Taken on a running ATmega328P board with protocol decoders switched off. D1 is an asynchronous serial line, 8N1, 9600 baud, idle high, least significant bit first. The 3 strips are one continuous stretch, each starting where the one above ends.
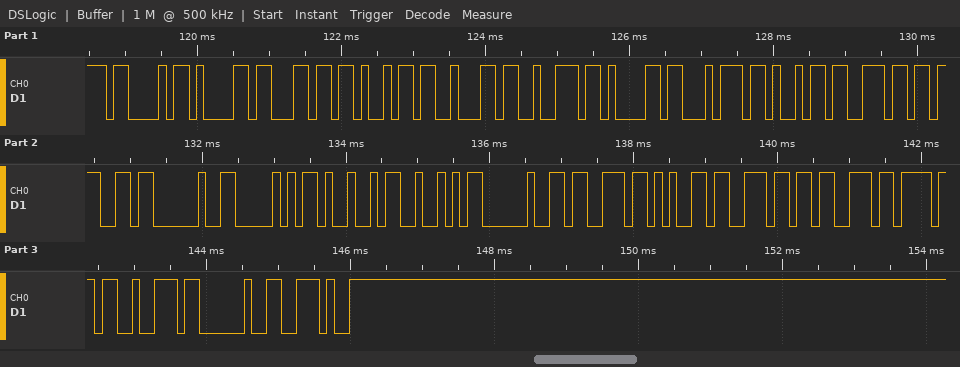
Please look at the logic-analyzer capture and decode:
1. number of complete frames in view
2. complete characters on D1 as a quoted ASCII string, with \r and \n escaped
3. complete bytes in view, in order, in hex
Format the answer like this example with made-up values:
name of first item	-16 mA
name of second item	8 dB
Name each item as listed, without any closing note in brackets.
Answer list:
number of complete frames in view	24
complete characters on D1 as a quoted ASCII string, with \r and \n escaped	"Calibrating PIR sensor ."
complete bytes in view, in order, in hex	43 61 6C 69 62 72 61 74 69 6E 67 20 50 49 52 20 73 65 6E 73 6F 72 20 2E
